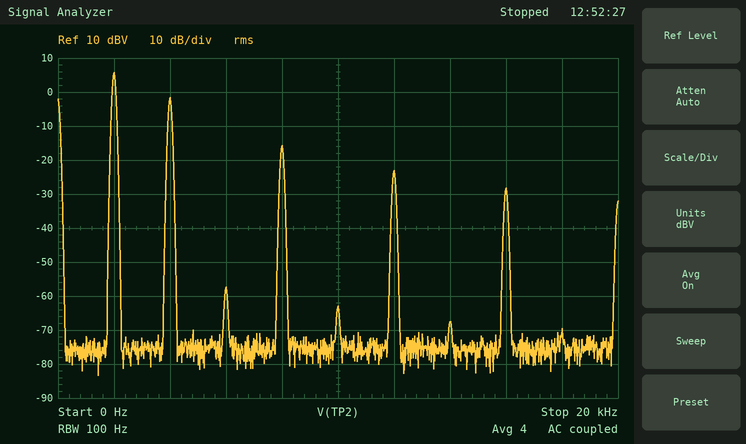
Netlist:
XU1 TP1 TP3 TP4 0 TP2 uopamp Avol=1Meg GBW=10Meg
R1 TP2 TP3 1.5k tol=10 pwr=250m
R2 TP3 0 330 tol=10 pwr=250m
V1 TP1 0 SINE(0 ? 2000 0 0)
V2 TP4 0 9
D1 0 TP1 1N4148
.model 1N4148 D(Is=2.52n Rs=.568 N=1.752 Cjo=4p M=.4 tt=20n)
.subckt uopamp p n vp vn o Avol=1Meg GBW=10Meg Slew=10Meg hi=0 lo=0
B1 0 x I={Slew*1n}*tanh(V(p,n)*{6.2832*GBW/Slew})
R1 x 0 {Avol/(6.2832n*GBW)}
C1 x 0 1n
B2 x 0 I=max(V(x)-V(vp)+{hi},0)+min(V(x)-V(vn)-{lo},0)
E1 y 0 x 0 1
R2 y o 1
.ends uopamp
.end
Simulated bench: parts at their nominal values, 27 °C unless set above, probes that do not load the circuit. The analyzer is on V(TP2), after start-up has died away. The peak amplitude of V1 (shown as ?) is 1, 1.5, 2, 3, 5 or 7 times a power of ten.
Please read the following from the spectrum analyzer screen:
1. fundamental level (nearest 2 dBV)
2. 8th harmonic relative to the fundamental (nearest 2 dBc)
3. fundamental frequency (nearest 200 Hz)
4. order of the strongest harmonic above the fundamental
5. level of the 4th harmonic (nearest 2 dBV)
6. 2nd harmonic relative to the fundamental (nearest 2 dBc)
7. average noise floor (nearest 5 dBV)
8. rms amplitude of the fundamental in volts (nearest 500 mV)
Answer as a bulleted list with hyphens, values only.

- 6 dBV
- -34 dBc
- 2.0 kHz
- 2
- -16 dBV
- -8 dBc
- -75 dBV
- 2.0 V
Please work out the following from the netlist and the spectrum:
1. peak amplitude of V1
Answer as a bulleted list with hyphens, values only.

- 1 V
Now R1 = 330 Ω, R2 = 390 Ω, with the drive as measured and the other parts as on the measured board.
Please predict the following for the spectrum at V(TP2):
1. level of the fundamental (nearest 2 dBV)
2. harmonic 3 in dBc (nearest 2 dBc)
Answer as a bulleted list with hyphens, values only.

- -4 dBV
- -54 dBc
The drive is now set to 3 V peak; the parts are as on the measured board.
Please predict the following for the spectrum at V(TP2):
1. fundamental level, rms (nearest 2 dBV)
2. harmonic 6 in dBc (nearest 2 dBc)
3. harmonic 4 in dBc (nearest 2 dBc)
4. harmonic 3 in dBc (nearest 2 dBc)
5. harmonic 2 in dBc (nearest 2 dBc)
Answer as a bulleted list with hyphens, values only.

- 12 dBV
- -20 dBc
- -14 dBc
- -14 dBc
- -12 dBc
